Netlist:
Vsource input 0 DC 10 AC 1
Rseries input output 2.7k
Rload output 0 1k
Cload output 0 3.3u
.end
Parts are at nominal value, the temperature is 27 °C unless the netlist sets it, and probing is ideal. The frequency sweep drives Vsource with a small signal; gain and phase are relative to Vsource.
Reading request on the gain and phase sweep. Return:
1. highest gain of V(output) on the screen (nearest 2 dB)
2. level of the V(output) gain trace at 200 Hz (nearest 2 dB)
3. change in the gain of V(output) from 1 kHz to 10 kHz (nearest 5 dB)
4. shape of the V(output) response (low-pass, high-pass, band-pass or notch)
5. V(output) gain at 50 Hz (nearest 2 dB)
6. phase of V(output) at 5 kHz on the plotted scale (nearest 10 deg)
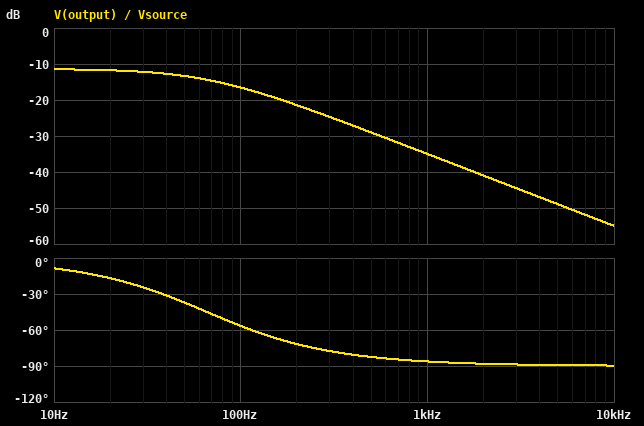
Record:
-12 dB
-22 dB
-20 dB
low-pass
-14 dB
-90 deg
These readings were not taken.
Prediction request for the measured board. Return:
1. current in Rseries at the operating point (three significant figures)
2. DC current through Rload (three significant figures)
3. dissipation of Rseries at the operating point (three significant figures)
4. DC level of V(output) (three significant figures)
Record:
2.70 mA
2.70 mA
19.7 mW
2.70 V
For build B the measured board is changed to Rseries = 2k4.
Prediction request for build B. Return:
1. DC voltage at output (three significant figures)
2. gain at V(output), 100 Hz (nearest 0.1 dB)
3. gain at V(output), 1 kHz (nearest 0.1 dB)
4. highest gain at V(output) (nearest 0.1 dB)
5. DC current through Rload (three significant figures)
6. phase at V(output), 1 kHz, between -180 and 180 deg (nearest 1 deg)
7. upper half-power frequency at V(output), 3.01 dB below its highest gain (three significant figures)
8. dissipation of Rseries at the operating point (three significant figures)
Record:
2.94 V
-15.6 dB
-34.0 dB
-10.6 dB
2.94 mA
-86 deg
68.3 Hz
20.8 mW
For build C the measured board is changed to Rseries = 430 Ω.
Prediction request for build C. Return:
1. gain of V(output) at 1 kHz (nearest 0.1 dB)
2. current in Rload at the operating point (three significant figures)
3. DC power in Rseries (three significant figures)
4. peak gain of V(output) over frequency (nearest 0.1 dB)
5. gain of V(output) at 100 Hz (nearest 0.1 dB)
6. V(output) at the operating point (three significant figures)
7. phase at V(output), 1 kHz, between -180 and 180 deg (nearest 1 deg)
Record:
-19.1 dB
6.99 mA
21.0 mW
-3.1 dB
-4.5 dB
6.99 V
-81 deg
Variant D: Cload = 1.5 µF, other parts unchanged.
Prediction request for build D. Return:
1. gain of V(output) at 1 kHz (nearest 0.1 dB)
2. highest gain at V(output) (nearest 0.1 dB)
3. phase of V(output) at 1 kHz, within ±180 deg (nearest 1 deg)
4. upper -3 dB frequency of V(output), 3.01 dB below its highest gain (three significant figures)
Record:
-28.2 dB
-11.4 dB
-82 deg
145 Hz
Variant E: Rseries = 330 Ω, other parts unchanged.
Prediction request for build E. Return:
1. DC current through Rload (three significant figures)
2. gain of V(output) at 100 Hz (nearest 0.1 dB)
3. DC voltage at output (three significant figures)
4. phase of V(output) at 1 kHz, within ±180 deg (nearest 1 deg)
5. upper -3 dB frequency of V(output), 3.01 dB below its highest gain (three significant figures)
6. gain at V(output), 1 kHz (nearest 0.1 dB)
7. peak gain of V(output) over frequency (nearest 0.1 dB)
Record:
7.52 mA
-3.5 dB
7.52 V
-79 deg
194 Hz
-16.9 dB
-2.5 dB
